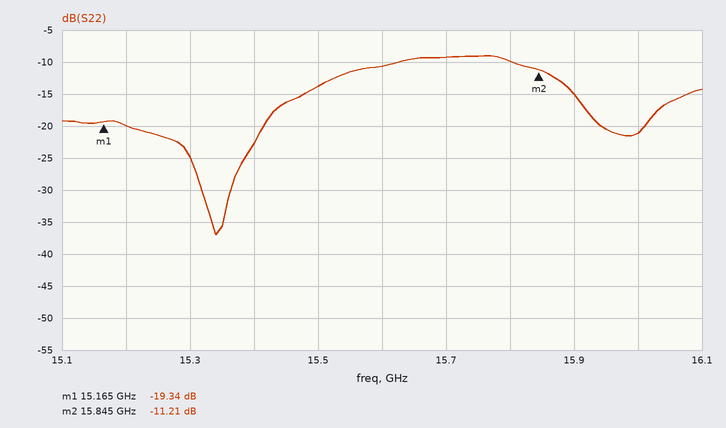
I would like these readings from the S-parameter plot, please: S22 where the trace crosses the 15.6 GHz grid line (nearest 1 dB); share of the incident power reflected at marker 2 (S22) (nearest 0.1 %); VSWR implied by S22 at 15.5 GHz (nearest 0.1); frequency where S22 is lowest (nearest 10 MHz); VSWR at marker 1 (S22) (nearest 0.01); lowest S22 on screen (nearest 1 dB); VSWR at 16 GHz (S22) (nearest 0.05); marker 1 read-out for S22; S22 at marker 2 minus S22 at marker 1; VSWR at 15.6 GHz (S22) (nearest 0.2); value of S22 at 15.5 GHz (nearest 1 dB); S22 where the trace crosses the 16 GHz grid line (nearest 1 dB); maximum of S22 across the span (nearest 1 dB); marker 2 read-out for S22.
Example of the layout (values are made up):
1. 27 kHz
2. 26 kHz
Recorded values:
1. -11 dB
2. 7.6 %
3. 1.5
4. 15.34 GHz
5. 1.24
6. -37 dB
7. 1.20
8. -19.34 dB
9. 8.13 dB
10. 1.8
11. -14 dB
12. -21 dB
13. -9 dB
14. -11.21 dB
